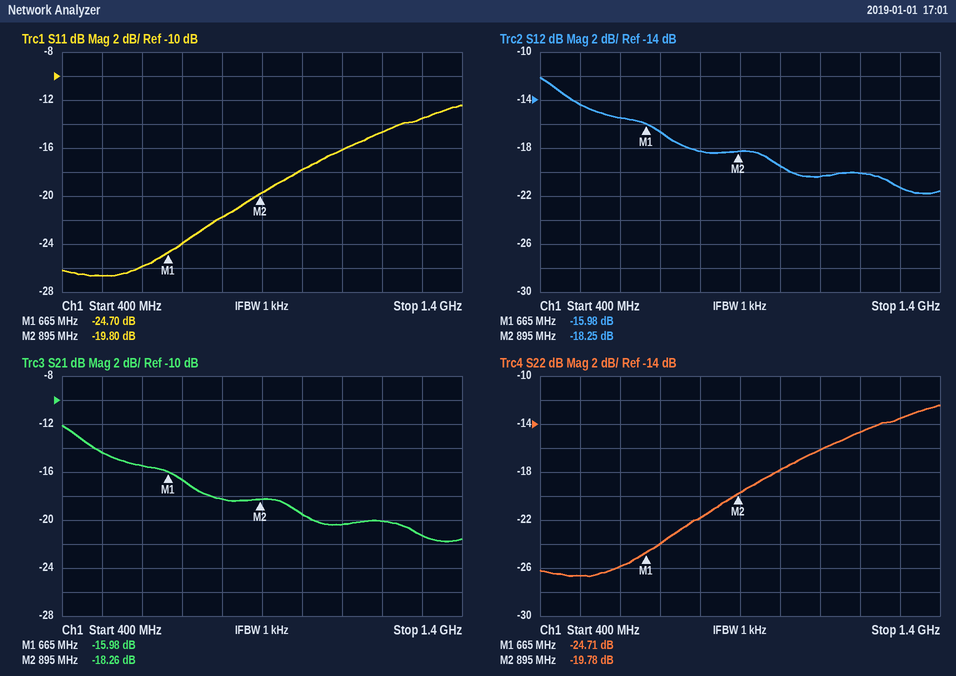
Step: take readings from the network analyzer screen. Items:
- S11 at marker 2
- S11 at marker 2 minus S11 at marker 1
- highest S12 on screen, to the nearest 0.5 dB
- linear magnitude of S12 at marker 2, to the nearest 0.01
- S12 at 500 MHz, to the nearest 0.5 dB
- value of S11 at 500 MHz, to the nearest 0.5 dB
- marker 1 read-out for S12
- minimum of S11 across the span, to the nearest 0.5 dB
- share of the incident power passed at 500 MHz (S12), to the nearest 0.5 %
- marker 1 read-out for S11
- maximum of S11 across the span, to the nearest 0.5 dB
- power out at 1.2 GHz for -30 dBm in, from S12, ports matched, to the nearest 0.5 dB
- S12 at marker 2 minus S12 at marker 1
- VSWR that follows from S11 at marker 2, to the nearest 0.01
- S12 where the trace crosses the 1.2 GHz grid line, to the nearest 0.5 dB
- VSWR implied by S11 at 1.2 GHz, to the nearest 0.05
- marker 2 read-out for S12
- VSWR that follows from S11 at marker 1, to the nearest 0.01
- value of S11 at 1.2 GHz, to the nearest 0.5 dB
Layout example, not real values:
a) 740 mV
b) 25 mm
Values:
a) -19.80 dB
b) 4.90 dB
c) -12.0 dB
d) 0.12
e) -14.5 dB
f) -26.5 dB
g) -15.98 dB
h) -26.5 dB
i) 3.5 %
j) -24.70 dB
k) -12.5 dB
l) -50.0 dBm
m) -2.27 dB
n) 1.23
o) -20.0 dB
p) 1.45
q) -18.25 dB
r) 1.12
s) -14.5 dB
